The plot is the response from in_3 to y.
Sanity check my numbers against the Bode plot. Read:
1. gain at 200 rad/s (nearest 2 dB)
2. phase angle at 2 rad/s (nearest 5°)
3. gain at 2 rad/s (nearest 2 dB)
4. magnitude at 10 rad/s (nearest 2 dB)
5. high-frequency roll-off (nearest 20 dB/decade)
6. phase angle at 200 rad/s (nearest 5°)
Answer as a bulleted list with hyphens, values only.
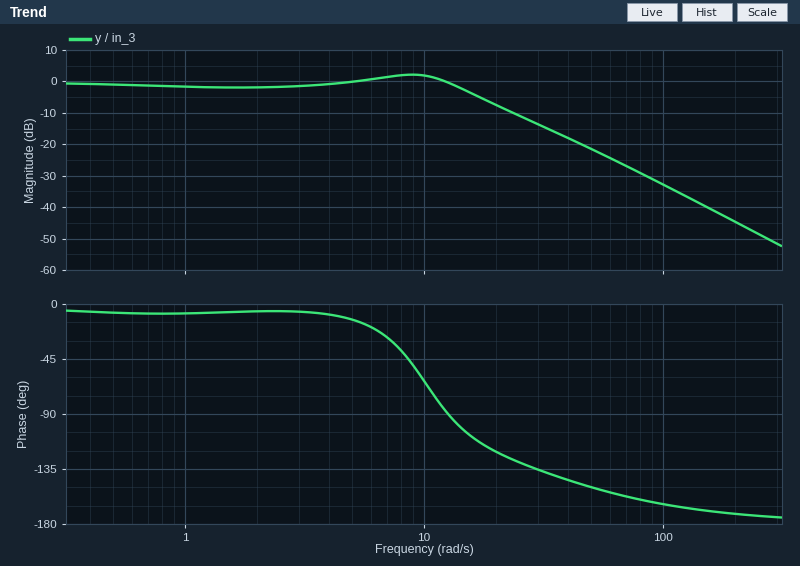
- -44 dB
- -5°
- -2 dB
- 2 dB
- -40 dB/decade
- -170°
